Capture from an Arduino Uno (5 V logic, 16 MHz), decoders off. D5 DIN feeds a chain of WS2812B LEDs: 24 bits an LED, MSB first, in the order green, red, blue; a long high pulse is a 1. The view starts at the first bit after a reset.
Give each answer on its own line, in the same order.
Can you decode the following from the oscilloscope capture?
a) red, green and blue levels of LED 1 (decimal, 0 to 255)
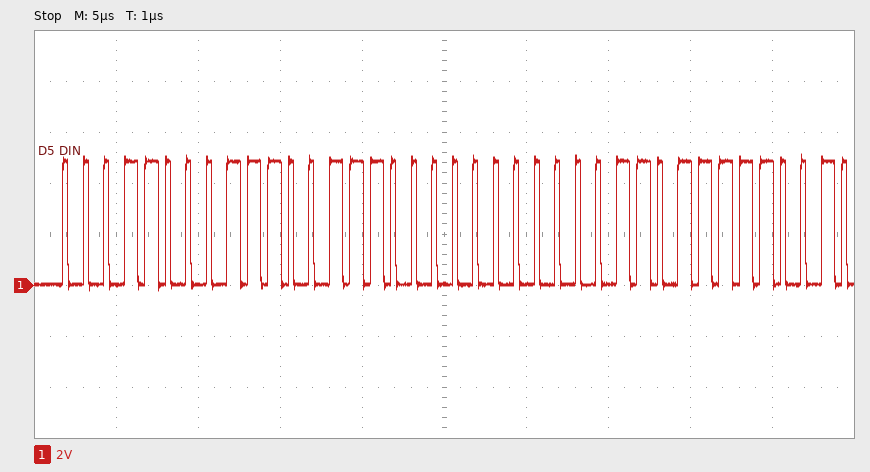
231, 24, 0
